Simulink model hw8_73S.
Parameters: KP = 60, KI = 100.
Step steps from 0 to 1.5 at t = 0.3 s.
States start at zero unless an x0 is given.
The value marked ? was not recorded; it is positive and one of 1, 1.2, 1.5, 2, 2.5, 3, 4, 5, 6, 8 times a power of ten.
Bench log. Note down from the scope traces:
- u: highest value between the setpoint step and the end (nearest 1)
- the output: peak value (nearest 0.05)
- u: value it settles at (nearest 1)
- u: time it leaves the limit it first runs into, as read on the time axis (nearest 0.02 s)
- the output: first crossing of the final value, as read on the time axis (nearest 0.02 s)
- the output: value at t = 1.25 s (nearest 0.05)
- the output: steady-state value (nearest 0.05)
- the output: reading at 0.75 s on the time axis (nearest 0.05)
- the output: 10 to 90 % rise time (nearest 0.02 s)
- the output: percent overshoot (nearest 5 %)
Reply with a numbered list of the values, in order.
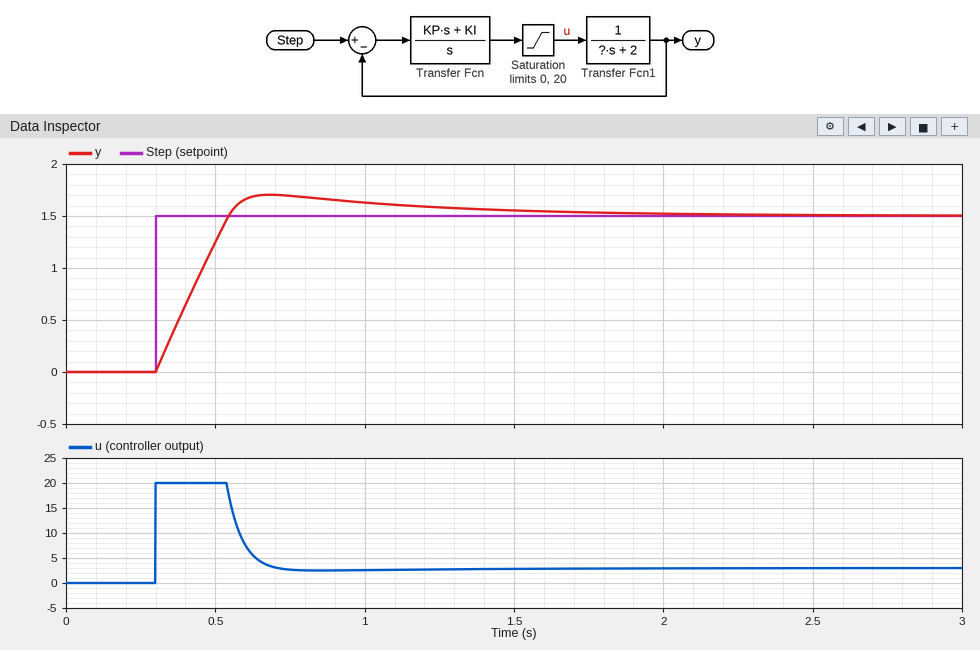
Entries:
1. 20
2. 1.70
3. 3
4. 0.54 s
5. 0.54 s
6. 1.60
7. 1.50
8. 1.70
9. 0.20 s
10. 15 %
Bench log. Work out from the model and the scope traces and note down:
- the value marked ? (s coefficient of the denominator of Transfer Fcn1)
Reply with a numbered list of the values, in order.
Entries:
1. 3
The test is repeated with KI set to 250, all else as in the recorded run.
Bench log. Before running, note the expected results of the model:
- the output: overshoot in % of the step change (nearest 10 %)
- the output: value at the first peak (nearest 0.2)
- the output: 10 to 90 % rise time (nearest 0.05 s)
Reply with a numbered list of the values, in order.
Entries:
1. 30 %
2. 2.0
3. 0.20 s
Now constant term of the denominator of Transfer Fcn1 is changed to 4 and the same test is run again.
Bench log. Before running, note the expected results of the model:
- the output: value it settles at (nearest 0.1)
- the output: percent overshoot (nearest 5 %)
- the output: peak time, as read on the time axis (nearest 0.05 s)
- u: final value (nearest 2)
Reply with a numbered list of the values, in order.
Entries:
1. 1.5
2. 10 %
3. 0.70 s
4. 6
